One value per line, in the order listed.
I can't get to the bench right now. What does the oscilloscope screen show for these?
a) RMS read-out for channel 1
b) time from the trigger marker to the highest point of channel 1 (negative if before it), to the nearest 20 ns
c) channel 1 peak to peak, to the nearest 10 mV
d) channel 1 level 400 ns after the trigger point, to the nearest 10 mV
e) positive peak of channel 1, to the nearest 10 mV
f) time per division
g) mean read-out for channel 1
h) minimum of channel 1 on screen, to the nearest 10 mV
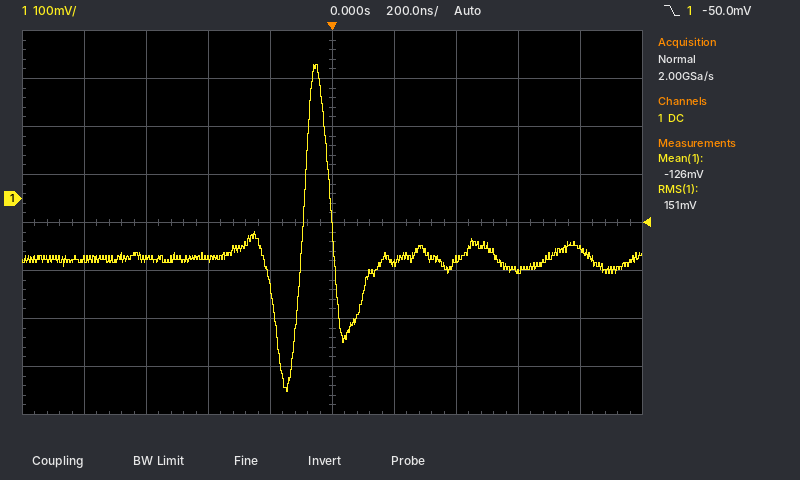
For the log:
151 mV
-60 ns
680 mV
-130 mV
280 mV
200 ns
-126 mV
-400 mV
